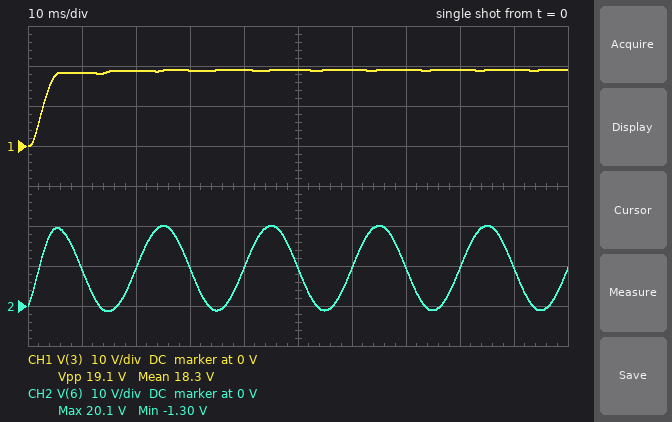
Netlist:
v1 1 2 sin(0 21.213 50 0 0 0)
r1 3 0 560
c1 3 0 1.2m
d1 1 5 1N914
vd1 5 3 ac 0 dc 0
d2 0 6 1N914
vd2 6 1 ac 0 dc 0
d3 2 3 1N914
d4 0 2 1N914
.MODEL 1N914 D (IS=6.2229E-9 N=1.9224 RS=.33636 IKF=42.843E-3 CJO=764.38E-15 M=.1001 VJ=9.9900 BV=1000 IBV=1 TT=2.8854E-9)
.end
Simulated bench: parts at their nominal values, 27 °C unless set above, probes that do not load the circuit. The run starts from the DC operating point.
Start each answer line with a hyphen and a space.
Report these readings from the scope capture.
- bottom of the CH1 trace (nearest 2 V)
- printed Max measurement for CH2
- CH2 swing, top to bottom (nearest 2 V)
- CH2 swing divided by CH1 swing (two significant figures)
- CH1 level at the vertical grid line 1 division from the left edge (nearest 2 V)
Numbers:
- 0 V
- 20.1 V
- 22 V
- 1.1
- 18 V
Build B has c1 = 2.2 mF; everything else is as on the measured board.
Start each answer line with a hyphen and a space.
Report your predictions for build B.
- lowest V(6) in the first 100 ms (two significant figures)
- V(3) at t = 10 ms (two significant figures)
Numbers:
- -1.8 V
- 17 V
